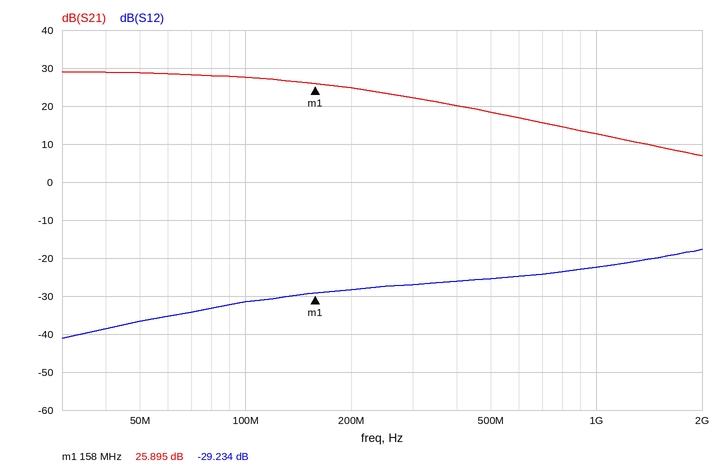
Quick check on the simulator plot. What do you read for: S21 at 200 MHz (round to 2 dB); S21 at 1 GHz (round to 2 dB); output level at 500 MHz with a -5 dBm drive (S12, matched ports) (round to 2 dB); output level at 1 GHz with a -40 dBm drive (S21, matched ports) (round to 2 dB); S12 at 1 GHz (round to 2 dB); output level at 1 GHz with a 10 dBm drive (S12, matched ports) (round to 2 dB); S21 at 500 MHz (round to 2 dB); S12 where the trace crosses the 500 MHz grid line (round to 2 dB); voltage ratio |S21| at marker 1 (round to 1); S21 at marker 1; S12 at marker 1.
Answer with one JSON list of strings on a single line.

["24 dB", "12 dB", "-30 dBm", "-28 dBm", "-22 dB", "-12 dBm", "18 dB", "-26 dB", "20", "25.895 dB", "-29.234 dB"]
